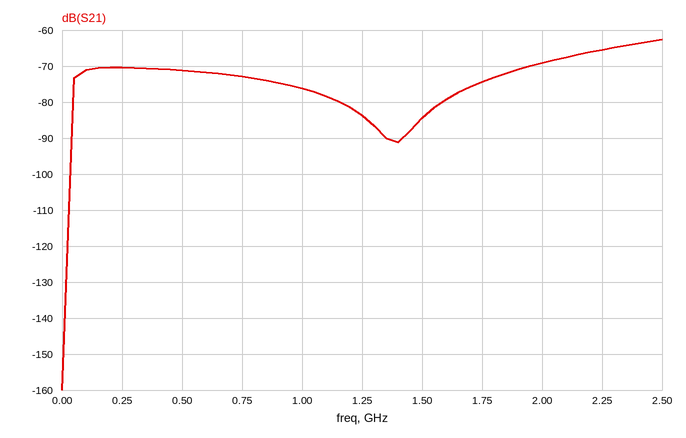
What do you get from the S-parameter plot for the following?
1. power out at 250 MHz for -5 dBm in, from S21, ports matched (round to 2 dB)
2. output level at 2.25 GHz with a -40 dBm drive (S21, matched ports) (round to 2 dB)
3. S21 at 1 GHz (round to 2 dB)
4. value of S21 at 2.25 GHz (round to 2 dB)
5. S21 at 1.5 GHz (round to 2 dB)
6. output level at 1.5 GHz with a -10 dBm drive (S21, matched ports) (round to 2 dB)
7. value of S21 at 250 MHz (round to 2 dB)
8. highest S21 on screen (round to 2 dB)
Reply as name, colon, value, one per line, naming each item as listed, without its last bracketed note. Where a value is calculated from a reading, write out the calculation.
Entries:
power out at 250 MHz for -5 dBm in, from S21, ports matched: -5 dBm + (-70 dB) = -76 dBm
output level at 2.25 GHz with a -40 dBm drive (S21, matched ports): -40 dBm + (-66 dB) = -106 dBm
S21 at 1 GHz: -76 dB
value of S21 at 2.25 GHz: -66 dB
S21 at 1.5 GHz: -84 dB
output level at 1.5 GHz with a -10 dBm drive (S21, matched ports): -10 dBm + (-84 dB) = -94 dBm
value of S21 at 250 MHz: -70 dB
highest S21 on screen: -62 dB
